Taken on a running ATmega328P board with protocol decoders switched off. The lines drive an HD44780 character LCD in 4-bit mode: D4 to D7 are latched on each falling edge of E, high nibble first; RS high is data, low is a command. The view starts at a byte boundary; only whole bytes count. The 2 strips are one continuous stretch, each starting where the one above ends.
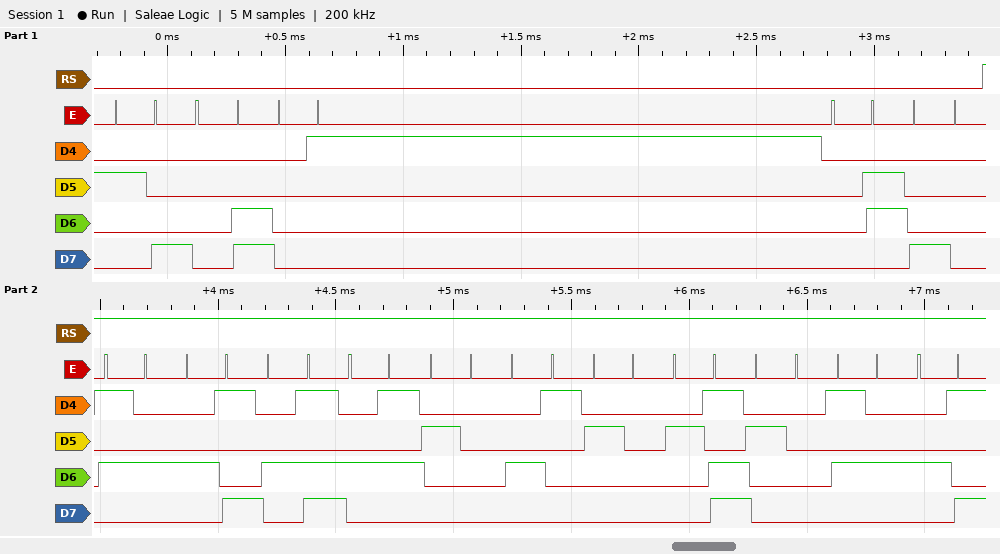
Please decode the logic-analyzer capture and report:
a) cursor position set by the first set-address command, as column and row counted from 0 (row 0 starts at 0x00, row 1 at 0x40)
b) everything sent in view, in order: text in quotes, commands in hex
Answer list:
column 0, row 0
0x28 0x0C 0x01 0x06 0x80 "TIME A - TI"
